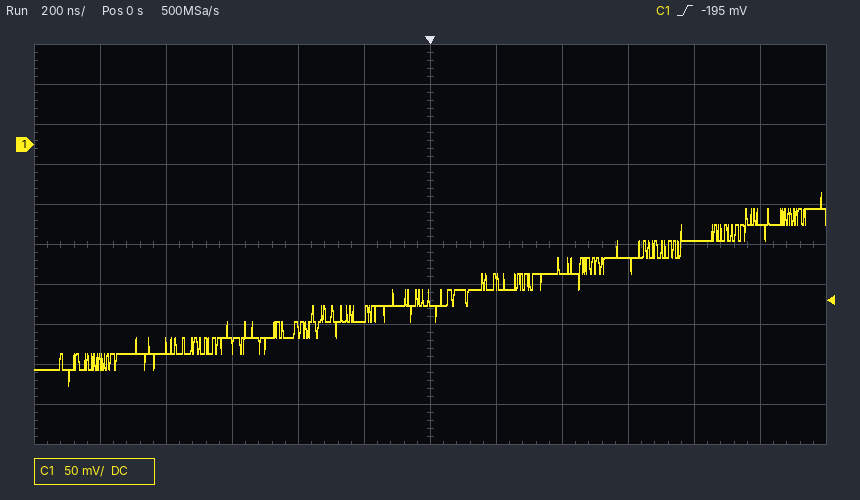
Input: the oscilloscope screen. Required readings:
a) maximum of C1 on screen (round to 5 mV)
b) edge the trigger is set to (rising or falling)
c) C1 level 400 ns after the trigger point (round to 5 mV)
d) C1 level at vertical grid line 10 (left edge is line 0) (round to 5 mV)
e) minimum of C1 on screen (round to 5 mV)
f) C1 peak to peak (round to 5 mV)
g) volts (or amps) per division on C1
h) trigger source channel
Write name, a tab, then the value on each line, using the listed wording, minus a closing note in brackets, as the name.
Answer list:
maximum of C1 on screen	-60 mV
edge the trigger is set to	rising
C1 level 400 ns after the trigger point	-160 mV
C1 level at vertical grid line 10 (left edge is line 0)	-120 mV
minimum of C1 on screen	-300 mV
C1 peak to peak	240 mV
volts (or amps) per division on C1	50 mV
trigger source channel	C1
